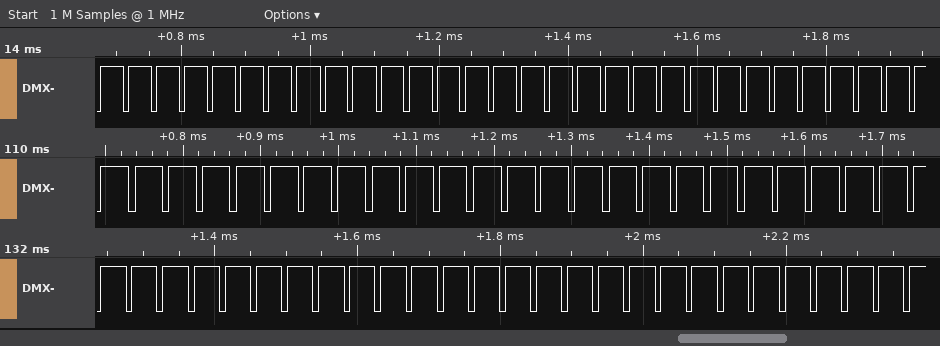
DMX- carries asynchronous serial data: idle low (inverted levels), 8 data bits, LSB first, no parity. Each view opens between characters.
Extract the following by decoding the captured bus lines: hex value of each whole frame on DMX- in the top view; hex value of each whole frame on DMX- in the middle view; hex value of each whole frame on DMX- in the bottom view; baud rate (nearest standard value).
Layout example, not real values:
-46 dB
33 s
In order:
08, 08, 08, 08, 08, 08, 08, 08, 08, 08, 08, 08, 08, 08
08, 08, 08, 08, 08, 08, 08, 08, 08, 08, 08, 08
08, 08, 08, 08, 08, 08, 08, 08, 08, 08, 08, 08, 08
115200 baud
